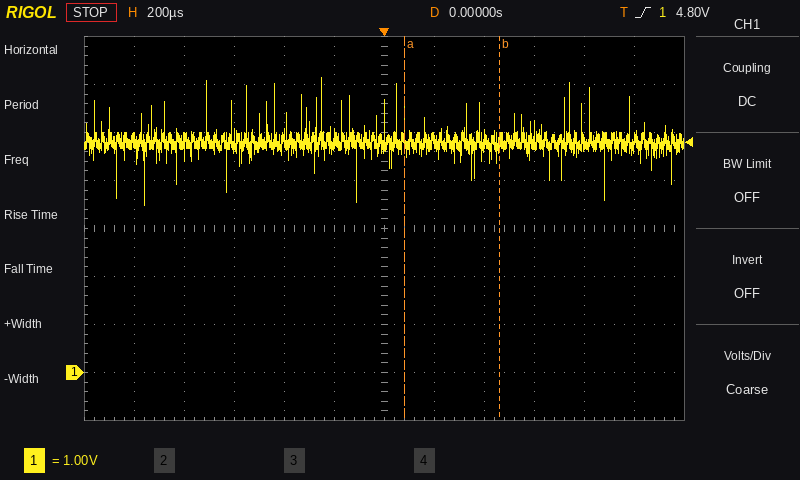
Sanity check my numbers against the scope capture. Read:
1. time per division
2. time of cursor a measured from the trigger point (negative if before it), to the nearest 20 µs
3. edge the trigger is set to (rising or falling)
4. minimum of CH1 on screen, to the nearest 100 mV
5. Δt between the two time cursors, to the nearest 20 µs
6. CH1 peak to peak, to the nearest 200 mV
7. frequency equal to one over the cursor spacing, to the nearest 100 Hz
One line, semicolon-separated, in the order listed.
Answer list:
200 µs; +80 µs; rising; 3.5 V; 380 µs; 2.6 V; 2.6 kHz
